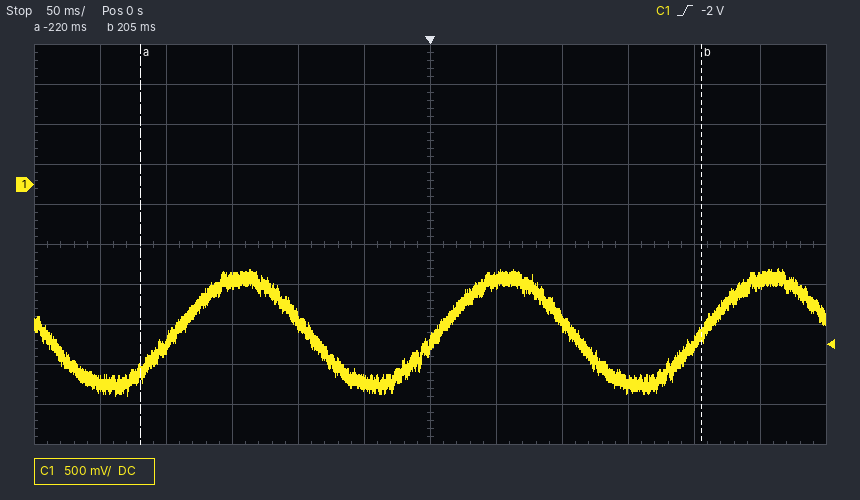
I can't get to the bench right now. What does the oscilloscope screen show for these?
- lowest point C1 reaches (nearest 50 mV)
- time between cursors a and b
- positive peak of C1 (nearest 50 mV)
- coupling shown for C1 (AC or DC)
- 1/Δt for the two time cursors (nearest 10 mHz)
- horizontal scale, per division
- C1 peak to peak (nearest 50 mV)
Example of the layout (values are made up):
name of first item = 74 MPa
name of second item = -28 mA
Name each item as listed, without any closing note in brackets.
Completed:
lowest point C1 reaches = -2.65 V
time between cursors a and b = 425 ms
positive peak of C1 = -1.05 V
coupling shown for C1 = DC
1/Δt for the two time cursors = 2.35 Hz
horizontal scale, per division = 50 ms
C1 peak to peak = 1.60 V
